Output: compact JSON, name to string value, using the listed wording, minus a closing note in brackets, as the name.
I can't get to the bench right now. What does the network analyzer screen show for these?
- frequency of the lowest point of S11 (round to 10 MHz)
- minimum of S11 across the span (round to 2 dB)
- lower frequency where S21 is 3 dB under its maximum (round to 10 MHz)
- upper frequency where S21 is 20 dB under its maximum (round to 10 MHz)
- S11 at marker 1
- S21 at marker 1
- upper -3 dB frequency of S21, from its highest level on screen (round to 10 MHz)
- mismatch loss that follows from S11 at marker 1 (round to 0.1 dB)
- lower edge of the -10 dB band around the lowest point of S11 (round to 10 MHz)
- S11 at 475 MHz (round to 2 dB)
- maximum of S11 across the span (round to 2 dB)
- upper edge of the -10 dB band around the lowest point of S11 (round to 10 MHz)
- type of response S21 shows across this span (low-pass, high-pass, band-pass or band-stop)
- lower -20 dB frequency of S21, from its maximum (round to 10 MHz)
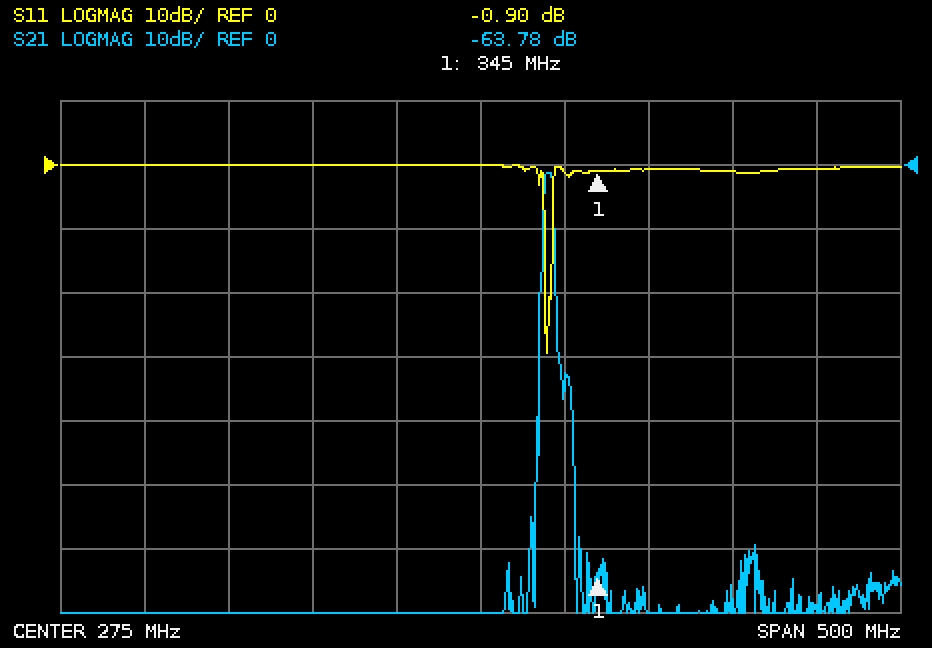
{"frequency of the lowest point of S11": "310 MHz", "minimum of S11 across the span": "-30 dB", "lower frequency where S21 is 3 dB under its maximum": "310 MHz", "upper frequency where S21 is 20 dB under its maximum": "320 MHz", "S11 at marker 1": "-0.90 dB", "S21 at marker 1": "-63.78 dB", "upper -3 dB frequency of S21, from its highest level on screen": "320 MHz", "mismatch loss that follows from S11 at marker 1": "7.3 dB", "lower edge of the -10 dB band around the lowest point of S11": "310 MHz", "S11 at 475 MHz": "0 dB", "maximum of S11 across the span": "0 dB", "upper edge of the -10 dB band around the lowest point of S11": "320 MHz", "type of response S21 shows across this span": "band-pass", "lower -20 dB frequency of S21, from its maximum": "310 MHz"}
